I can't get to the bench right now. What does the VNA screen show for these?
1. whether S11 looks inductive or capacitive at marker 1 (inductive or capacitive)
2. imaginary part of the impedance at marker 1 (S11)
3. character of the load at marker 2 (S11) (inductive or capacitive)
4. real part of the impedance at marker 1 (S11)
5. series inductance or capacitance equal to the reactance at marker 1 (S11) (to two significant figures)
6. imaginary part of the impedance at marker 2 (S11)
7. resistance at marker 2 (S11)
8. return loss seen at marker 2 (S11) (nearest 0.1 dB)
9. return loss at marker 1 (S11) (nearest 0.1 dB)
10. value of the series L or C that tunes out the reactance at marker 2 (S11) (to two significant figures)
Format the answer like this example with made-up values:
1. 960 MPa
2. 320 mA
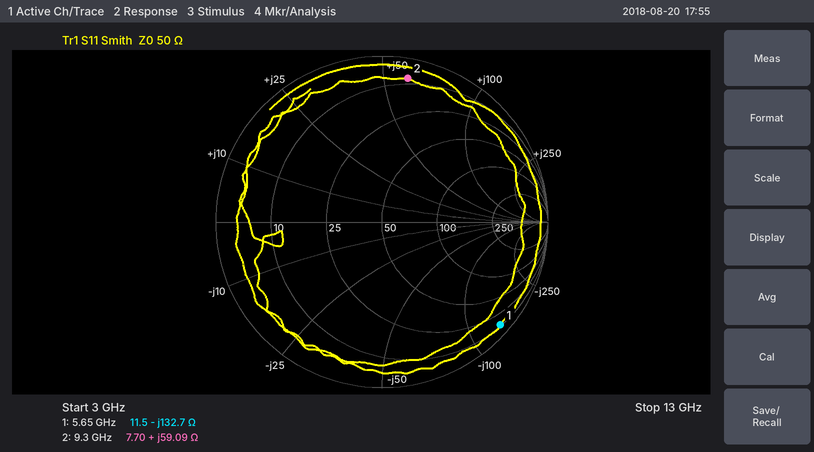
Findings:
1. capacitive
2. -132.7 Ω
3. inductive
4. 11.5 Ω
5. 210 fF
6. +59.09 Ω
7. 7.70 Ω
8. 1.1 dB
9. 0.5 dB
10. 290 fF
